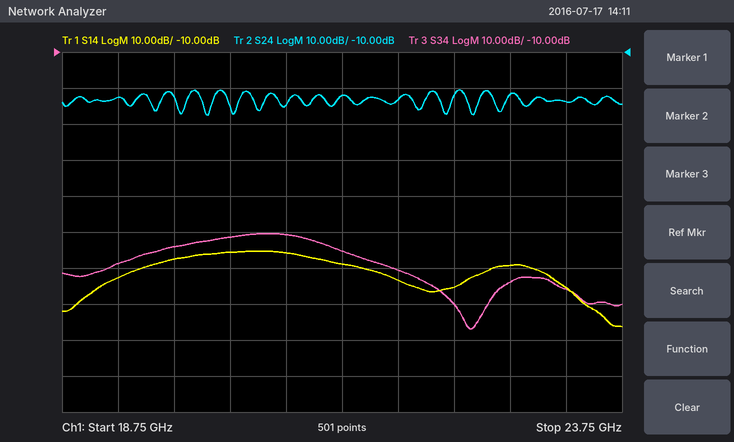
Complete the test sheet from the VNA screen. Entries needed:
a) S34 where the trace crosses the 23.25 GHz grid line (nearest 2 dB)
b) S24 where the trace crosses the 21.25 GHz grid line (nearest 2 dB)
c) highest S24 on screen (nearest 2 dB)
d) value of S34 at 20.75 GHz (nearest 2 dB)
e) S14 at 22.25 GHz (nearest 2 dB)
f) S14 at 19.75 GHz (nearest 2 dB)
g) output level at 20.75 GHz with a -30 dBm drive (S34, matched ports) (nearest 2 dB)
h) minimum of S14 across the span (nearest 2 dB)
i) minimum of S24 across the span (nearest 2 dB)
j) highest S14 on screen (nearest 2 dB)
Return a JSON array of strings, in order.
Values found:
["-76 dB", "-22 dB", "-20 dB", "-60 dB", "-76 dB", "-68 dB", "-90 dBm", "-86 dB", "-28 dB", "-66 dB"]
